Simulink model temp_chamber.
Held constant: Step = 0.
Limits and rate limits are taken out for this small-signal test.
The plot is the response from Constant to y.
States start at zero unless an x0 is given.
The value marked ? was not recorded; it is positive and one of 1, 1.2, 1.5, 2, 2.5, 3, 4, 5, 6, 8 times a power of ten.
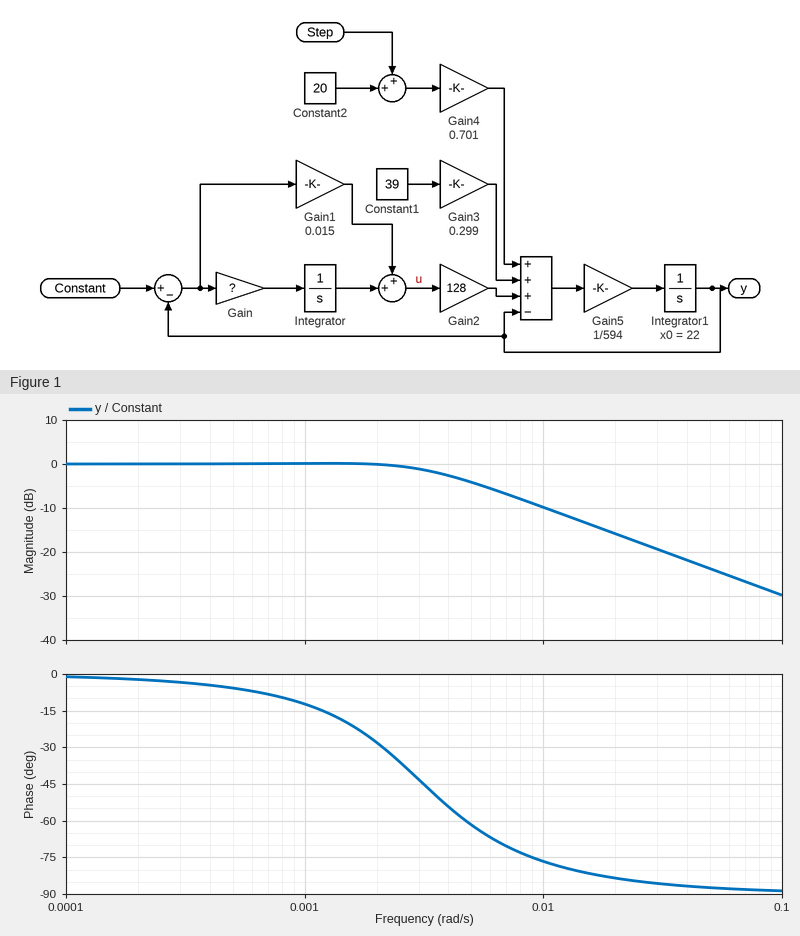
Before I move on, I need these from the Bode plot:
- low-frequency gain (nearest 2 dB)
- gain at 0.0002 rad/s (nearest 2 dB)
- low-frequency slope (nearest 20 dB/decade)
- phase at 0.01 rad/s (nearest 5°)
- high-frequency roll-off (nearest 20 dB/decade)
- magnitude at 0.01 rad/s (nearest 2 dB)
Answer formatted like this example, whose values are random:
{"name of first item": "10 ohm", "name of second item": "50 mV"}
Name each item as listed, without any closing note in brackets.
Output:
{"low-frequency gain": "0 dB", "gain at 0.0002 rad/s": "0 dB", "low-frequency slope": "0 dB/decade", "phase at 0.01 rad/s": "-75°", "high-frequency roll-off": "-20 dB/decade", "magnitude at 0.01 rad/s": "-10 dB"}
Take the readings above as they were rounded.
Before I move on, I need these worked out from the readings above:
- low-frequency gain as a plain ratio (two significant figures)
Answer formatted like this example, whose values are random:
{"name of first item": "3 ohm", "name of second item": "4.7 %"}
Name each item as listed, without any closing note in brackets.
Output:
{"low-frequency gain as a plain ratio": "1.0"}
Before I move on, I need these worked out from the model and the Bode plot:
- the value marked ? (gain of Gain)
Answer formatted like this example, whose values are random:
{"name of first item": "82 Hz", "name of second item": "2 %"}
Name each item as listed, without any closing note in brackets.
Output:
{"the value marked ?": "4e-05"}
